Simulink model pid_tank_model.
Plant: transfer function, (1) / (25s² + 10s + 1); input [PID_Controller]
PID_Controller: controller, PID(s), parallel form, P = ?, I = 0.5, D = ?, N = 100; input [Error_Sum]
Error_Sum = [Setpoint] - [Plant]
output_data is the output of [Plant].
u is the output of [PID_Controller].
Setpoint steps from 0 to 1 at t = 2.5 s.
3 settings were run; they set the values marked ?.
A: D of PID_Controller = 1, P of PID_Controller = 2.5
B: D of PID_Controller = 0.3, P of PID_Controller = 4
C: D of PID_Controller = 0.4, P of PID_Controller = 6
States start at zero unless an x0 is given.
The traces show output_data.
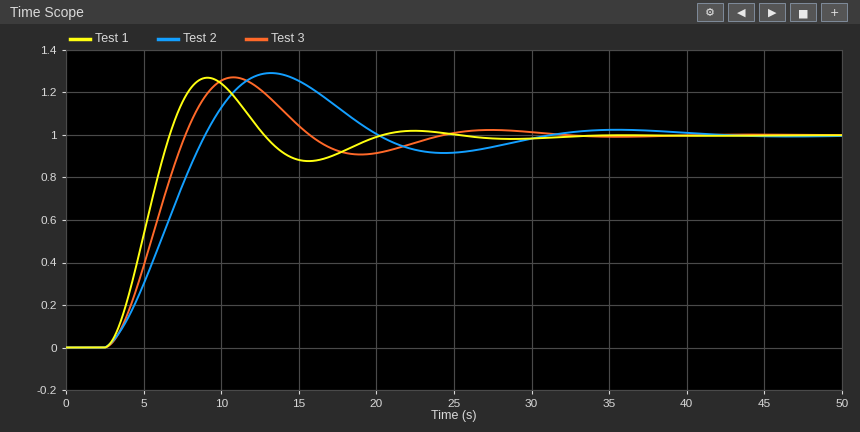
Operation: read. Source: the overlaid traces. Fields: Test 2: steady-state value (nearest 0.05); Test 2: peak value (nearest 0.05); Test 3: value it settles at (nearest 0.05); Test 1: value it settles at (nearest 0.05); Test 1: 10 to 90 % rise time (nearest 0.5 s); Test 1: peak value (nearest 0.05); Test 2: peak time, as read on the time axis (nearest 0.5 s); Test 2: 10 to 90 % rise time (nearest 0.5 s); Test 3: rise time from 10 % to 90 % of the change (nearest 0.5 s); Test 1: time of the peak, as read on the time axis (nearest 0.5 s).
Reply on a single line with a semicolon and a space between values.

1.00; 1.30; 1.00; 1.00; 3.0 s; 1.25; 13.0 s; 4.5 s; 3.5 s; 9.0 s
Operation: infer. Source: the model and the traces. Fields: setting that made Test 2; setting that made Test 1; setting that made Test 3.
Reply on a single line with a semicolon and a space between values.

A; C; B
